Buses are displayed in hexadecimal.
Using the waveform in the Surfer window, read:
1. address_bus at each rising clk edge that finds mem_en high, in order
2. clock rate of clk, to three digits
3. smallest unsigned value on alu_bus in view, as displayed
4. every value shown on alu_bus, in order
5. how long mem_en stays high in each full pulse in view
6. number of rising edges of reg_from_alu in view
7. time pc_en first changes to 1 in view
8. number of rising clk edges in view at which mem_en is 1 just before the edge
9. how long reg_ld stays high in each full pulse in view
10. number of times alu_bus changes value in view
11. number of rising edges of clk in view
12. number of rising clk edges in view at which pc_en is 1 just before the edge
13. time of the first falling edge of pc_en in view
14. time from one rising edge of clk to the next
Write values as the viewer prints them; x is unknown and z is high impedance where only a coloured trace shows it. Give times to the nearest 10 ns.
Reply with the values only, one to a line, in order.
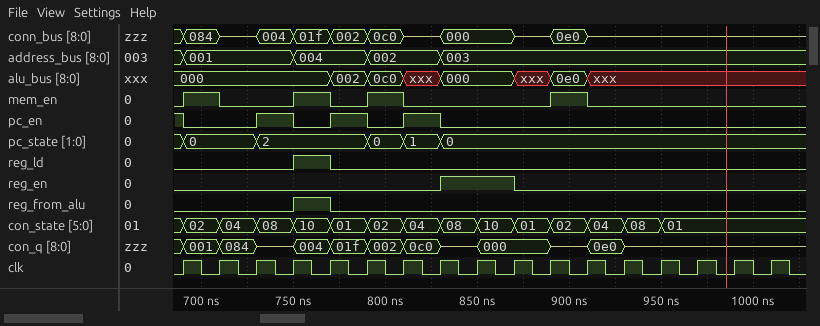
001, 004, 002, 003
50.0 MHz
000
000, 002, 0c0, xxx, 000, xxx, 0e0, xxx
20 ns, 20 ns, 20 ns, 20 ns
1
730 ns
4
20 ns
7
17
4
690 ns
20 ns
